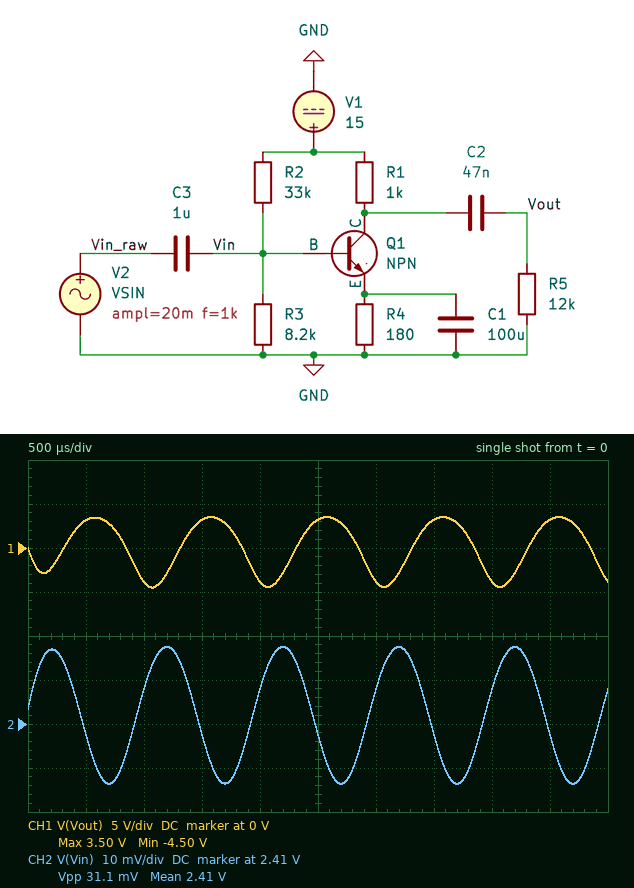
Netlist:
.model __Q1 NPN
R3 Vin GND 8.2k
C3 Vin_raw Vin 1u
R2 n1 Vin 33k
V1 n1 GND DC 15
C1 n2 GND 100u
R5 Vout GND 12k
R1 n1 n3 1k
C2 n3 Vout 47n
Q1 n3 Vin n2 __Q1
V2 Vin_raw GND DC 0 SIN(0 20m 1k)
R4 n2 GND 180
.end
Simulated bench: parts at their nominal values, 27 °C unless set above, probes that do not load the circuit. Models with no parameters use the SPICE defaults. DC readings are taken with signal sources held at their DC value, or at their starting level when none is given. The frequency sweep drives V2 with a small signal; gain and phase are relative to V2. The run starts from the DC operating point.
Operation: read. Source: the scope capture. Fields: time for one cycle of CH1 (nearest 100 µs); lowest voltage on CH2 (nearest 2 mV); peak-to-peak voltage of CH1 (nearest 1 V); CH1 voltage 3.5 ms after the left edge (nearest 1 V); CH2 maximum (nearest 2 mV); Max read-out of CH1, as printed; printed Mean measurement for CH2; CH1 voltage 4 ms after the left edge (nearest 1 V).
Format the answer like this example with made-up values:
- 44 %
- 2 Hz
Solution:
- 1.0 ms
- 2.396 V
- 8 V
- 3 V
- 2.428 V
- 3.50 V
- 2.41 V
- -4 V
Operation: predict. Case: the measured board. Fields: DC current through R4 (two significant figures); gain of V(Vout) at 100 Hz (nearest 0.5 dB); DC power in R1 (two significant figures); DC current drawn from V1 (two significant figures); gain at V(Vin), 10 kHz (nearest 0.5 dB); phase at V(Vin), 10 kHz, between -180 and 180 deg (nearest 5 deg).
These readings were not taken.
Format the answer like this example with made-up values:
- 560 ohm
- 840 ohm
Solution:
- 8.8 mA
- 20.0 dB
- 76 mW
- 9.1 mA
- 0 dB
- 5 deg
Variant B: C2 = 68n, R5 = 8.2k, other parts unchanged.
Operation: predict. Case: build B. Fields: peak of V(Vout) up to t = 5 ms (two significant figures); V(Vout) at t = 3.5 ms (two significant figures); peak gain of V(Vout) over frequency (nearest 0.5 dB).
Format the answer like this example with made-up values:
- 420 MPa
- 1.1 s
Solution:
- 3.4 V
- 3.1 V
- 49.5 dB
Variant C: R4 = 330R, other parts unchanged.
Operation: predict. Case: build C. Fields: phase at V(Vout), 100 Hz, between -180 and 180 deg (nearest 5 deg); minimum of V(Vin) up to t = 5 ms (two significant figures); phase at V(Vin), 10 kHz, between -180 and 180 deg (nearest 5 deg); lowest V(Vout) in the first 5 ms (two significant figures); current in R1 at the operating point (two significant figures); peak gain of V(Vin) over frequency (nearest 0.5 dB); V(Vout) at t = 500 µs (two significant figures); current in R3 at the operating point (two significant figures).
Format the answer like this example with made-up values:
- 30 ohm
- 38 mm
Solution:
- -25 deg
- 2.6 V
- 0 deg
- -3.5 V
- 5.4 mA
- 0 dB
- 2.2 V
- 320 µA
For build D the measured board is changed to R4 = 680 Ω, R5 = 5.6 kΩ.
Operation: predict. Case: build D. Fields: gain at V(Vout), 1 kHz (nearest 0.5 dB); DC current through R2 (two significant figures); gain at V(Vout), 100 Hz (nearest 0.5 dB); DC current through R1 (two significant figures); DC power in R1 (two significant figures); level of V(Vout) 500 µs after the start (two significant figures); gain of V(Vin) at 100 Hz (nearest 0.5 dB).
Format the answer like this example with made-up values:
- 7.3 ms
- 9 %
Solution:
- 38.0 dB
- 370 µA
- 13.5 dB
- 2.9 mA
- 8.4 mW
- 1.2 V
- -5.5 dB
